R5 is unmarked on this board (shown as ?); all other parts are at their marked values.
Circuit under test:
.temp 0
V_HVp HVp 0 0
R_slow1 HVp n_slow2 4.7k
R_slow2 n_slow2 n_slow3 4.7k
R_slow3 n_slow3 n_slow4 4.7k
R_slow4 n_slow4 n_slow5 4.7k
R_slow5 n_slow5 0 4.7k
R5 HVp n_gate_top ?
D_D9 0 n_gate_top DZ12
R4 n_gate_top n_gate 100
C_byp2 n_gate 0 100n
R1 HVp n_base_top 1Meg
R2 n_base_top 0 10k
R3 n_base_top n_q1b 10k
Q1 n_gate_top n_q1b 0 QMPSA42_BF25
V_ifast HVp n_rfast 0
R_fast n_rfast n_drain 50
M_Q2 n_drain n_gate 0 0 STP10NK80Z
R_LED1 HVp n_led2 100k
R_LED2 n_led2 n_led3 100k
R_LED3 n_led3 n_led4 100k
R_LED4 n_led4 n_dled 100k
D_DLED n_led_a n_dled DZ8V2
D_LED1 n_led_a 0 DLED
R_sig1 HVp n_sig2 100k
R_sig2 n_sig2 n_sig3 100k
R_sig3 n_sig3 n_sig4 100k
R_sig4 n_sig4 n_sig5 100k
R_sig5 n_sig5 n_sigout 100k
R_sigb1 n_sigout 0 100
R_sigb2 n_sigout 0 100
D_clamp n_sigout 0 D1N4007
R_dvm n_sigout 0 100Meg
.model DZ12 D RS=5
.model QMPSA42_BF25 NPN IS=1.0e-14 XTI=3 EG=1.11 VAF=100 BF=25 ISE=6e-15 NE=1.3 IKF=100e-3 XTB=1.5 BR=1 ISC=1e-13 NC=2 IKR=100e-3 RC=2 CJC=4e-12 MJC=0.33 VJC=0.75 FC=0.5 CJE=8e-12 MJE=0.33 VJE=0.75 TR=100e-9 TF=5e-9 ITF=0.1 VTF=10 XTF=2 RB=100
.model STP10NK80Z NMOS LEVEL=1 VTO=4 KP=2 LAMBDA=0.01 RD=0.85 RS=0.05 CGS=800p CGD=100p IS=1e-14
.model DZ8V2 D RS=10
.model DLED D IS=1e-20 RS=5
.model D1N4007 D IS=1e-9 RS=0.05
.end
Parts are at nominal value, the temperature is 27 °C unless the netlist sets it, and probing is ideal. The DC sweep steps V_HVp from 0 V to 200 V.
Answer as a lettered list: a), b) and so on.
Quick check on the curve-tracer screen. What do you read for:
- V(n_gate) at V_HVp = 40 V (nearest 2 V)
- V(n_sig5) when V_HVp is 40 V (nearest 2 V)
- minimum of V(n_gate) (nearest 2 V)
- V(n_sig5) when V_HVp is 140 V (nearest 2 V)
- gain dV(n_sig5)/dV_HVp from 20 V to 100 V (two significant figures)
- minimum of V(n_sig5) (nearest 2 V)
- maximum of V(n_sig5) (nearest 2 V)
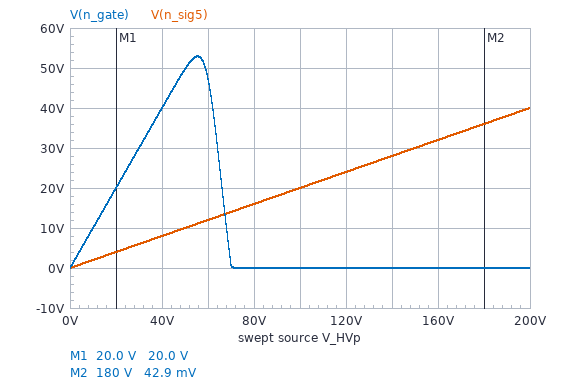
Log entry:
a) 40 V
b) 8 V
c) 0 V
d) 28 V
e) 0.20 V/V
f) 0 V
g) 40 V
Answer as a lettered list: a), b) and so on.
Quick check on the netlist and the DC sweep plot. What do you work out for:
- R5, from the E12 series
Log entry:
a) 1.2 MΩ
